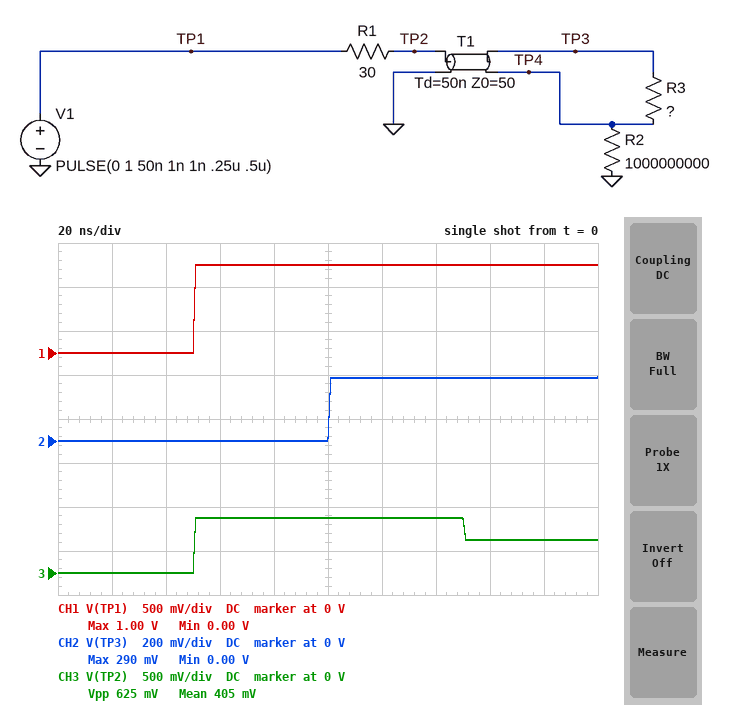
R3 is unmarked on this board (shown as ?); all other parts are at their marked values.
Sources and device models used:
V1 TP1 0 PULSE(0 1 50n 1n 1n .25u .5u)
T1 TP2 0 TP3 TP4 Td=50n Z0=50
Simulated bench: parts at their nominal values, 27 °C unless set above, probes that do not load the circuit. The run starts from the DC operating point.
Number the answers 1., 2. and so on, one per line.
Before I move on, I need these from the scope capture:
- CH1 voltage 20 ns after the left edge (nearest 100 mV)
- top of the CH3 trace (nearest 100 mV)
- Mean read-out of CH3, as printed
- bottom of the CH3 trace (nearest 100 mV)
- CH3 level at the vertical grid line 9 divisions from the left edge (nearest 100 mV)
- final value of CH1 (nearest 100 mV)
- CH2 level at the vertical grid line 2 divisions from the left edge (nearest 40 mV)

1. 0 V
2. 600 mV
3. 405 mV
4. 0 V
5. 400 mV
6. 1.0 V
7. 0 V
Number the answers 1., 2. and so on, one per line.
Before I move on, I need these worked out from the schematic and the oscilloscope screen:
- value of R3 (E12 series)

1. 15 Ω
